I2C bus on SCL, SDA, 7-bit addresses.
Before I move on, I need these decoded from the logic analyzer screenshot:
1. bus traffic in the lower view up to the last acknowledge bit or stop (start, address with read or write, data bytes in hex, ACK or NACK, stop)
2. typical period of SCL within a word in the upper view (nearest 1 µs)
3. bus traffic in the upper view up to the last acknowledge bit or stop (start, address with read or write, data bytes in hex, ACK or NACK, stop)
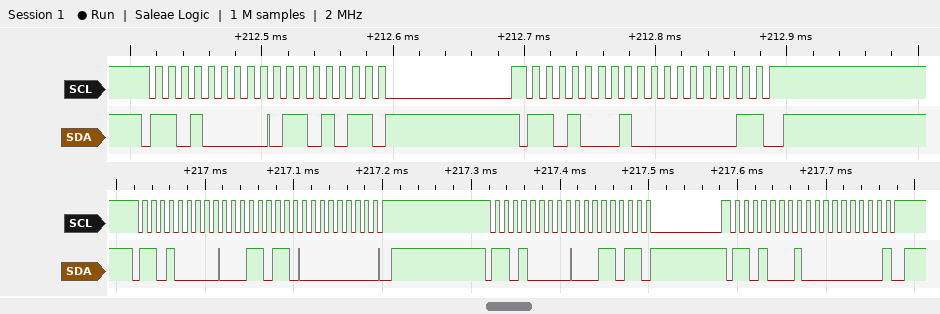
start, address 68 write ACK, 1B ACK, 00 ACK, stop, start, address 68 write ACK, 1B ACK, repeated start, address 68 read ACK, 00 NACK, stop
10 µs
start, address 68 write ACK, 6B ACK, repeated start, address 68 read ACK, 01 NACK, stop
